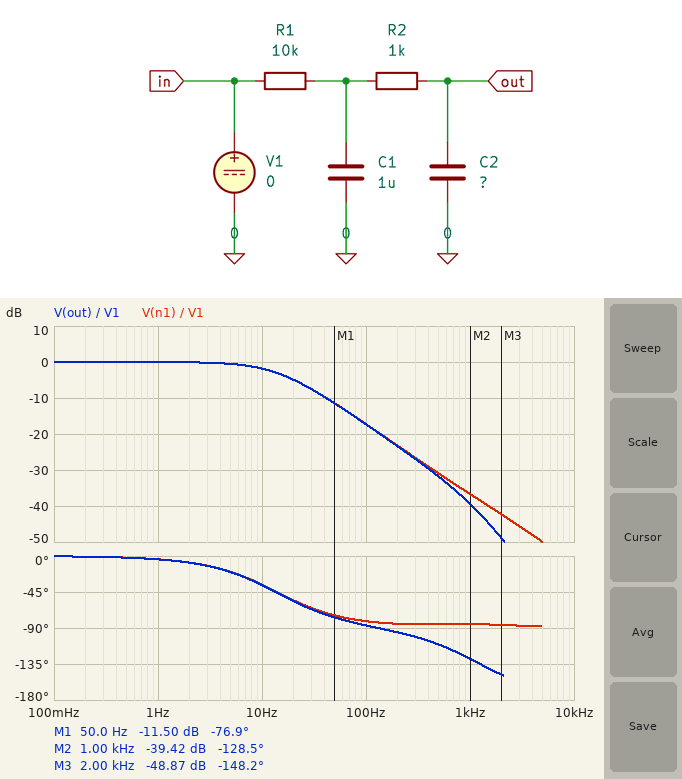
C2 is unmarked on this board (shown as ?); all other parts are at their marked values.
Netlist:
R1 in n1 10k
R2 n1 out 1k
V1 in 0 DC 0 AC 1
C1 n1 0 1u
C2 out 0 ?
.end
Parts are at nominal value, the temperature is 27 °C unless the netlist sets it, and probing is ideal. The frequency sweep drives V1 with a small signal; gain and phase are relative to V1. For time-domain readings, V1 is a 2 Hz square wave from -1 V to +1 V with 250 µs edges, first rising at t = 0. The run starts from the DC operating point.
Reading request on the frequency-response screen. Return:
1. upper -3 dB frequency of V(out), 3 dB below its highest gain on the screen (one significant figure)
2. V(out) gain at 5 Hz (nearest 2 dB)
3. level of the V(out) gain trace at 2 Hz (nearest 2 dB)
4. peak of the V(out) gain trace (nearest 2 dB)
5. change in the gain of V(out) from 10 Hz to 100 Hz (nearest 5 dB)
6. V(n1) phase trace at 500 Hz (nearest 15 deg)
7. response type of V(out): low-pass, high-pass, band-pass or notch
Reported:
10 Hz
0 dB
0 dB
0 dB
-15 dB
-90 deg
low-pass
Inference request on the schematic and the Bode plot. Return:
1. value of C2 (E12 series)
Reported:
150 nF
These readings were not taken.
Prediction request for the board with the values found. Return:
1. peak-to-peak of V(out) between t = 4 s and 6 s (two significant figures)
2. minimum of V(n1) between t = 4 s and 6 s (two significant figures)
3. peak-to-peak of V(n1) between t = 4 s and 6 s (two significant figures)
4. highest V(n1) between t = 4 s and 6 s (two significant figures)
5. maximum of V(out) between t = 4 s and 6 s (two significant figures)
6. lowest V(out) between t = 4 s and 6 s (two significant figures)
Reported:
2.0 V
-1.0 V
2.0 V
1.0 V
1.0 V
-1.0 V
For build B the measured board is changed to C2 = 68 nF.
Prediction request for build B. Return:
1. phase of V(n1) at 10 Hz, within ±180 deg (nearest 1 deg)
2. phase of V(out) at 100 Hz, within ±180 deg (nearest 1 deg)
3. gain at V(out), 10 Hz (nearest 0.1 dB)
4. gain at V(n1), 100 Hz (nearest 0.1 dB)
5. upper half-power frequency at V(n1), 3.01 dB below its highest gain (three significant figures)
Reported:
-34 deg
-84 deg
-1.6 dB
-16.6 dB
14.9 Hz
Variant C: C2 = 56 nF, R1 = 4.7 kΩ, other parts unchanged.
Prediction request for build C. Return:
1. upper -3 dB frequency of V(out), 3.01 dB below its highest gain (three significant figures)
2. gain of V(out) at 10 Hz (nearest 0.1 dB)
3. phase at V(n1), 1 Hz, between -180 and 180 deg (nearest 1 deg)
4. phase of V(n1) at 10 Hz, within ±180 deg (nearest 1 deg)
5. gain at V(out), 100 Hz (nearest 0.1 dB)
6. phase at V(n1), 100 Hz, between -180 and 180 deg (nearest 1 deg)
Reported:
32.0 Hz
-0.4 dB
-2 deg
-17 deg
-10.3 dB
-72 deg
